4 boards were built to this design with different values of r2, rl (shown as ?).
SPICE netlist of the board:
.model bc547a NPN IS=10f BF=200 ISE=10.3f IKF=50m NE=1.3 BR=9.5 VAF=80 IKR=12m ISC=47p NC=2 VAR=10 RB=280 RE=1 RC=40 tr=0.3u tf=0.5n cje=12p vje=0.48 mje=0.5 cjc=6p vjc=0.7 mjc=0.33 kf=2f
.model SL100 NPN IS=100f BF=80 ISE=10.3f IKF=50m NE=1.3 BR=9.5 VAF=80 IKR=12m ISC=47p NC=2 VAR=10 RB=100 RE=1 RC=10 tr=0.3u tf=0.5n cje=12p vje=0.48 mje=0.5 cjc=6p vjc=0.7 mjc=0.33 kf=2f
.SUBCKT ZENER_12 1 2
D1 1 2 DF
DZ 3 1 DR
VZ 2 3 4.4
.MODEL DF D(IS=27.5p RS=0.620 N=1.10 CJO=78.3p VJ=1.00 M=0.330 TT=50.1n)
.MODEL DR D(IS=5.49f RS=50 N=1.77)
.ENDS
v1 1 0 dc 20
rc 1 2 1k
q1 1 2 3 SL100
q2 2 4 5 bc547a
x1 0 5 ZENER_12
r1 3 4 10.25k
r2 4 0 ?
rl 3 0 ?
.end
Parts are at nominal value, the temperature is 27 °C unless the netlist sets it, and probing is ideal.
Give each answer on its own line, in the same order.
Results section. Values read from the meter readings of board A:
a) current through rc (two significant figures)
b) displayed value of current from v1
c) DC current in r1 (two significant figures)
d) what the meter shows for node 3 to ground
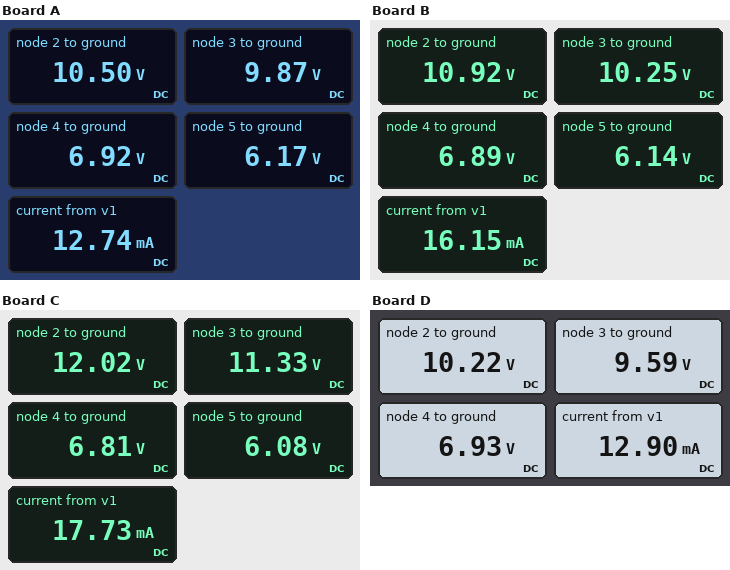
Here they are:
9.5 mA
12.74 mA
290 µA
9.87 V
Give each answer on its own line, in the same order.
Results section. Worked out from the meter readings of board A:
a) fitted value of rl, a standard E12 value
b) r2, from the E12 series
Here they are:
3.3 kΩ
33 kΩ
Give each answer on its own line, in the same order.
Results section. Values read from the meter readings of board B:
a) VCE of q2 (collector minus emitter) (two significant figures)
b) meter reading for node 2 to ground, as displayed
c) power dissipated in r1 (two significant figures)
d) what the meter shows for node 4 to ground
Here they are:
4.8 V
10.92 V
1.1 mW
6.89 V
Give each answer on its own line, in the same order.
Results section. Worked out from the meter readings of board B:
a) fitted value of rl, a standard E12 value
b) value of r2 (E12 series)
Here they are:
1.5 kΩ
27 kΩ
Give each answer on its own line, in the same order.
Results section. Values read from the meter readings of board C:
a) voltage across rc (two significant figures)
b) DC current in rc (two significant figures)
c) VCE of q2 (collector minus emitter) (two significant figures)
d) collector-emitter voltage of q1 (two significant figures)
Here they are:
8.0 V
8.0 mA
5.9 V
8.7 V
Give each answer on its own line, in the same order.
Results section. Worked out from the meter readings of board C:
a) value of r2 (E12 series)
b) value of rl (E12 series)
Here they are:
18 kΩ
1.2 kΩ
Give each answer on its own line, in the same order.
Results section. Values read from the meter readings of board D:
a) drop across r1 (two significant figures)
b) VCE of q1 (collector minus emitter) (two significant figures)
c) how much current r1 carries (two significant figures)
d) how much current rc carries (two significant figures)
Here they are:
2.7 V
10 V
260 µA
9.8 mA
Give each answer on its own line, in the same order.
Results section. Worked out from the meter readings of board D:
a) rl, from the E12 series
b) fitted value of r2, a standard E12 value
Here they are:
3.3 kΩ
39 kΩ
